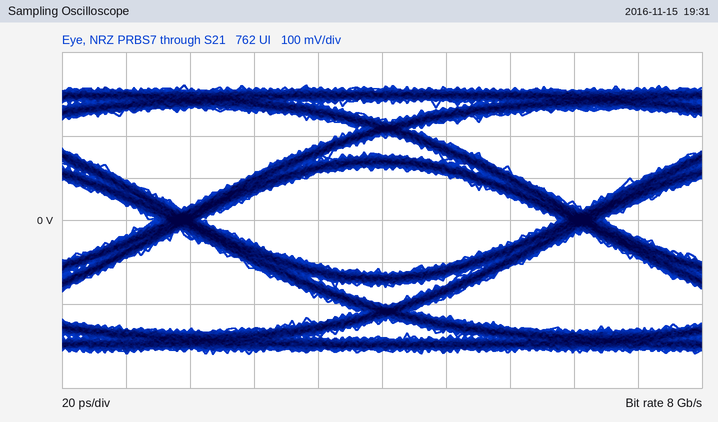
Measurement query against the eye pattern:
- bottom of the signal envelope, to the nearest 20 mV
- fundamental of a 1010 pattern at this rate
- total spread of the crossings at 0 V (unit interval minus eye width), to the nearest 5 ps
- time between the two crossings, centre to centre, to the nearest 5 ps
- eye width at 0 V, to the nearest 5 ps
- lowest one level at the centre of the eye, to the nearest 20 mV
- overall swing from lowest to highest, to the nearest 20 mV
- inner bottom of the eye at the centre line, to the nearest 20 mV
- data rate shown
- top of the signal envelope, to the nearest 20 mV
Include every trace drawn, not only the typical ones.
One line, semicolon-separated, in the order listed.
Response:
-320 mV; 4 GHz; 15 ps; 125 ps; 110 ps; 120 mV; 640 mV; -120 mV; 8 Gb/s; 320 mV
